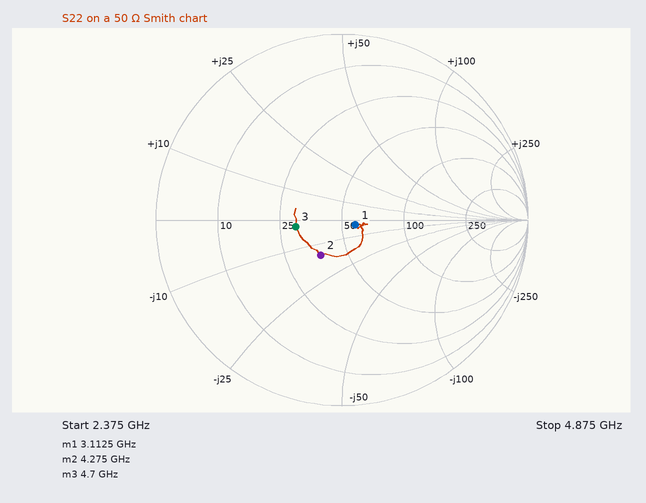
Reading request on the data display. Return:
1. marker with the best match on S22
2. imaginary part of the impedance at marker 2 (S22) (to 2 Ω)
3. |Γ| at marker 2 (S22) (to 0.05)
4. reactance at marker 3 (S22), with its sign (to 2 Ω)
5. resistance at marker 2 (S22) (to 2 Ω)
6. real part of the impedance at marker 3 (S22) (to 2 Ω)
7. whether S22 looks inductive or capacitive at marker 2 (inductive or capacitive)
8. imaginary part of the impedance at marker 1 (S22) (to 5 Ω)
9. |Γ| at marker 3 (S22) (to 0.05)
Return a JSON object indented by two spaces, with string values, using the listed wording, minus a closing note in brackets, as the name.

{
  "marker with the best match on S22": "marker 1",
  "imaginary part of the impedance at marker 2 (S22)": "-14 Ω",
  "|Γ| at marker 2 (S22)": "0.20",
  "reactance at marker 3 (S22), with its sign": "-2 Ω",
  "resistance at marker 2 (S22)": "38 Ω",
  "real part of the impedance at marker 3 (S22)": "30 Ω",
  "whether S22 looks inductive or capacitive at marker 2": "capacitive",
  "imaginary part of the impedance at marker 1 (S22)": "-5 Ω",
  "|Γ| at marker 3 (S22)": "0.25"
}
